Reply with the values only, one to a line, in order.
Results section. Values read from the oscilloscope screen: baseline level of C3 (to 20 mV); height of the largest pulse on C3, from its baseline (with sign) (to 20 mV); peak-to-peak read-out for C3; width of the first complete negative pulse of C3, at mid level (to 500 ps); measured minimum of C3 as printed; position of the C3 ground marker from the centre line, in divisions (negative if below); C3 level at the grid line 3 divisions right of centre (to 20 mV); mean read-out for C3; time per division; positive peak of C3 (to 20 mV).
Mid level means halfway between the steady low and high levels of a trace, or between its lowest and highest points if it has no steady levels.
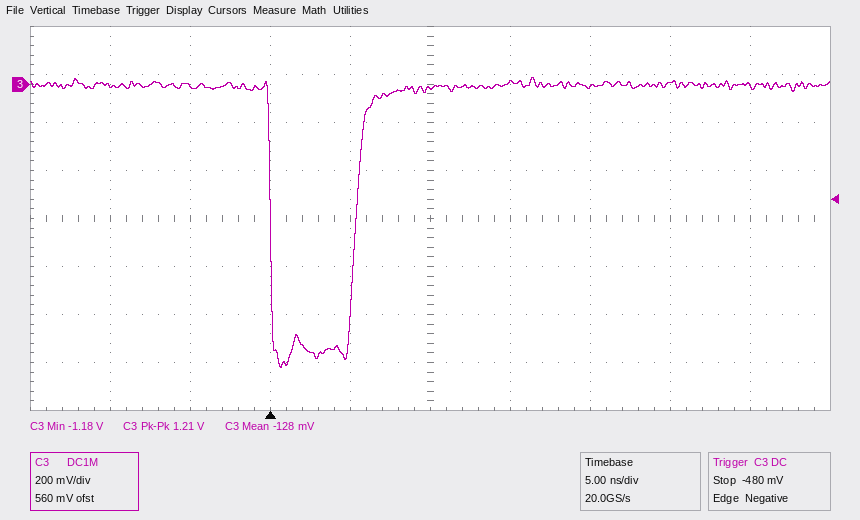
0 mV
-1.18 V
1.21 V
5.5 ns
-1.18 V
+2.8 div
0 mV
-128 mV
5 ns
20 mV
